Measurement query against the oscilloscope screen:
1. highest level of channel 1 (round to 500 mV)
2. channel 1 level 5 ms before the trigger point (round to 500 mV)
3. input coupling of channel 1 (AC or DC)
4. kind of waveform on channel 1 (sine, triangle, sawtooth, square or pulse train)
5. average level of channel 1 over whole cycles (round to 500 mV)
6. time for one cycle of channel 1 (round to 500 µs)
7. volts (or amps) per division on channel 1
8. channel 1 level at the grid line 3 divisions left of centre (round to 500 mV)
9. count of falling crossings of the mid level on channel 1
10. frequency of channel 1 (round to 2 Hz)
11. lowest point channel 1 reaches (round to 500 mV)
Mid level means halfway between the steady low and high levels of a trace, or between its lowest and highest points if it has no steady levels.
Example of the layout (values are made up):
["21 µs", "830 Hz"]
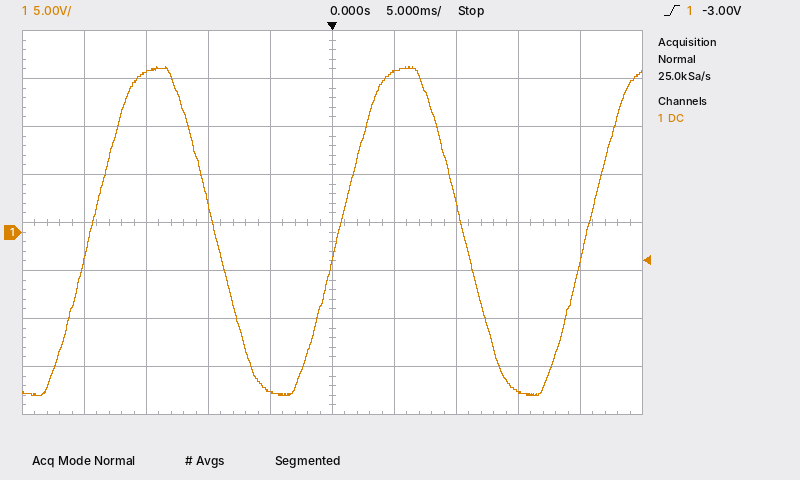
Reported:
["17.0 V", "-16.5 V", "DC", "sine", "0.0 V", "20.0 ms", "5 V", "16.5 V", "2", "50 Hz", "-17.0 V"]
